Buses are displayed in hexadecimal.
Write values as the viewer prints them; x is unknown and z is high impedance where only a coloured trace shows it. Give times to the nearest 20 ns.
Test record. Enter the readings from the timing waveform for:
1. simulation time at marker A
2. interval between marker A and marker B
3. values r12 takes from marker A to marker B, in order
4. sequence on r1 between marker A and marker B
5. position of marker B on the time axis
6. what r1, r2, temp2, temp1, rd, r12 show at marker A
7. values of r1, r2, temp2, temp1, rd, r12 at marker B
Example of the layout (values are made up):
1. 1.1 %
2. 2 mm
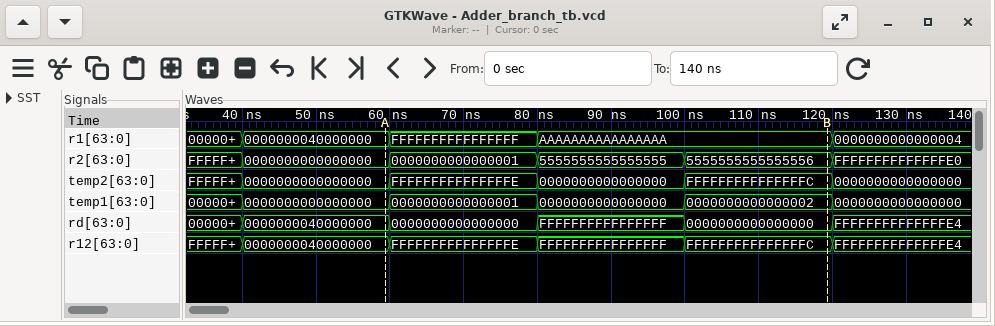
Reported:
1. 60 ns
2. 60 ns
3. 0000000040000000, FFFFFFFFFFFFFFFE, FFFFFFFFFFFFFFFF, FFFFFFFFFFFFFFFC
4. 0000000040000000, FFFFFFFFFFFFFFFF, AAAAAAAAAAAAAAAA
5. 120 ns
6. r1=0000000040000000, r2=0000000000000000, temp2=0000000000000000, temp1=0000000000000000, rd=0000000040000000, r12=0000000040000000
7. r1=AAAAAAAAAAAAAAAA, r2=5555555555555556, temp2=FFFFFFFFFFFFFFFC, temp1=0000000000000002, rd=0000000000000000, r12=FFFFFFFFFFFFFFFC
